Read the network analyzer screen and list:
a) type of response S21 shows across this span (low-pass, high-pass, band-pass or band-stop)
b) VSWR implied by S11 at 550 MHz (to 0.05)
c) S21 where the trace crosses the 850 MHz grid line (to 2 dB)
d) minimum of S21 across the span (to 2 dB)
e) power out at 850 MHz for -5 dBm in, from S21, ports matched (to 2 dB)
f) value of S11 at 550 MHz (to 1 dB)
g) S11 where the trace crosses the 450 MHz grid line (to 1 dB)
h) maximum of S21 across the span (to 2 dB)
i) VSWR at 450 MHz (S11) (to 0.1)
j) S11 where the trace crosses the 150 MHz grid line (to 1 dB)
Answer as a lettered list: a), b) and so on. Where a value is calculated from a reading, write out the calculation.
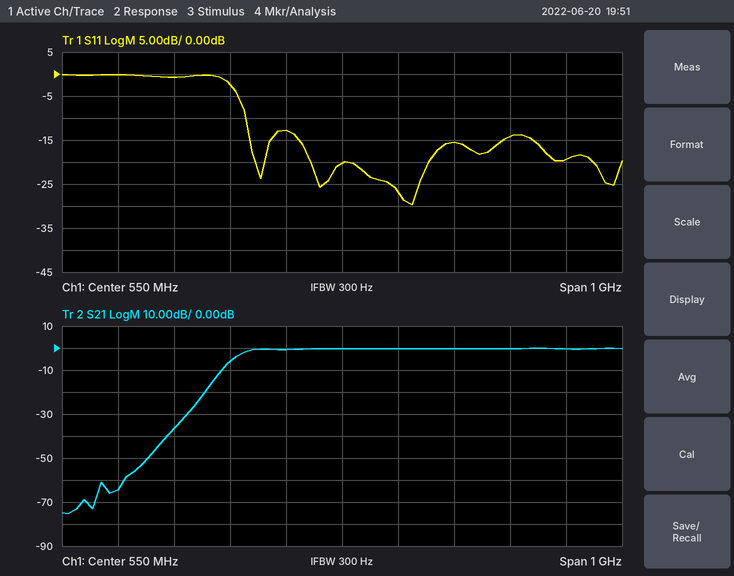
a) high-pass
b) |Γ| = 10^(-20/20) = 0.1000; VSWR = (1 + 0.1000)/(1 − 0.1000) ≈ 1.22, so 1.20 to the nearest 0.05
c) 0 dB
d) -76 dB
e) -5 dBm + (0 dB) = -6 dBm
f) -20 dB
g) -13 dB
h) 0 dB
i) |Γ| = 10^(-13/20) = 0.2239; VSWR = (1 + 0.2239)/(1 − 0.2239) ≈ 1.6
j) 0 dB
